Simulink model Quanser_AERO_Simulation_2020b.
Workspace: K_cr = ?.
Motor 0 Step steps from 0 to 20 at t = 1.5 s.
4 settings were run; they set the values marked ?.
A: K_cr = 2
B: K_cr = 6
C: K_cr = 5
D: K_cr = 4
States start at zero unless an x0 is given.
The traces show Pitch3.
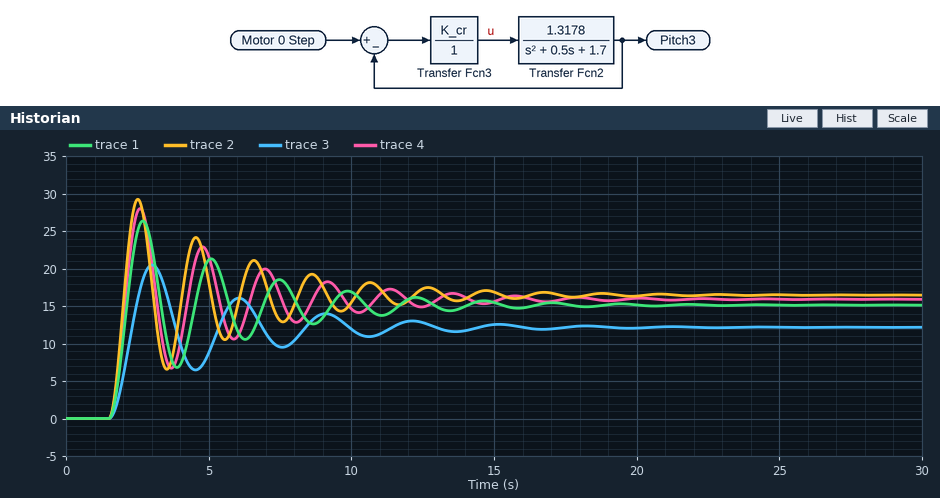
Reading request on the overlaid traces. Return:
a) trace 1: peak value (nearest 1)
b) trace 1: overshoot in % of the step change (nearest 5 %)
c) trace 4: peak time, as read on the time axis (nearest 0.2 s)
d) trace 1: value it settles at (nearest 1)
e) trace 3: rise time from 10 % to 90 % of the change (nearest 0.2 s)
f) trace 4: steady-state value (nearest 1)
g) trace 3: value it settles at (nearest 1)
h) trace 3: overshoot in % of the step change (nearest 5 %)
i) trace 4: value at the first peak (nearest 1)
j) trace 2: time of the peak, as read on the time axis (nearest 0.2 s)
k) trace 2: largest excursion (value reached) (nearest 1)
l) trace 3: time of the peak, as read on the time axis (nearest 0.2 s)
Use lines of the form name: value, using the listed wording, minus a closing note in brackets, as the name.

trace 1: peak value: 26
trace 1: overshoot in % of the step change: 75 %
trace 4: peak time, as read on the time axis: 2.6 s
trace 1: value it settles at: 15
trace 3: rise time from 10 % to 90 % of the change: 0.6 s
trace 4: steady-state value: 16
trace 3: value it settles at: 12
trace 3: overshoot in % of the step change: 70 %
trace 4: value at the first peak: 28
trace 2: time of the peak, as read on the time axis: 2.6 s
trace 2: largest excursion (value reached): 29
trace 3: time of the peak, as read on the time axis: 3.0 s
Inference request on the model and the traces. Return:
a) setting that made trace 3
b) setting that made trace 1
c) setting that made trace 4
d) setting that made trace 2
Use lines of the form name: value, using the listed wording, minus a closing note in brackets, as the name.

setting that made trace 3: A
setting that made trace 1: D
setting that made trace 4: C
setting that made trace 2: B
